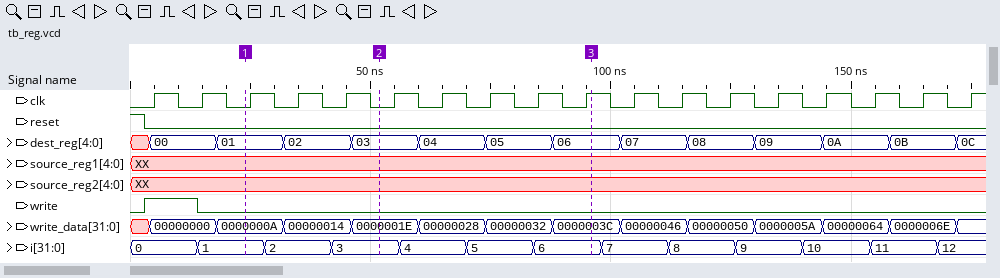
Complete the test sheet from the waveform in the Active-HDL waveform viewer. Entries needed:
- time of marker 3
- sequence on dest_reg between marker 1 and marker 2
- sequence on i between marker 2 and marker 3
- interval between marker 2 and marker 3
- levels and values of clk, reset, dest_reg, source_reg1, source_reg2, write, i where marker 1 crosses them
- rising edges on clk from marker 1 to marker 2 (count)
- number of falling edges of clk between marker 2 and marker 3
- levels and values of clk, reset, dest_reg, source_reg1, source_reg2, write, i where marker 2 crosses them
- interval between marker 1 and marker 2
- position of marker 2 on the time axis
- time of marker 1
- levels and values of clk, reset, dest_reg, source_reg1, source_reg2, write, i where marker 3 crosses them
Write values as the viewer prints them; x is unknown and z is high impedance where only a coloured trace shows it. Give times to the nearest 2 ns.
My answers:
96 ns
01, 02, 03
3, 4, 5, 6
44 ns
clk=0, reset=0, dest_reg=01, source_reg1=XX, source_reg2=XX, write=0, i=1
3
4
clk=0, reset=0, dest_reg=03, source_reg1=XX, source_reg2=XX, write=0, i=3
28 ns
52 ns
24 ns
clk=1, reset=0, dest_reg=06, source_reg1=XX, source_reg2=XX, write=0, i=6
